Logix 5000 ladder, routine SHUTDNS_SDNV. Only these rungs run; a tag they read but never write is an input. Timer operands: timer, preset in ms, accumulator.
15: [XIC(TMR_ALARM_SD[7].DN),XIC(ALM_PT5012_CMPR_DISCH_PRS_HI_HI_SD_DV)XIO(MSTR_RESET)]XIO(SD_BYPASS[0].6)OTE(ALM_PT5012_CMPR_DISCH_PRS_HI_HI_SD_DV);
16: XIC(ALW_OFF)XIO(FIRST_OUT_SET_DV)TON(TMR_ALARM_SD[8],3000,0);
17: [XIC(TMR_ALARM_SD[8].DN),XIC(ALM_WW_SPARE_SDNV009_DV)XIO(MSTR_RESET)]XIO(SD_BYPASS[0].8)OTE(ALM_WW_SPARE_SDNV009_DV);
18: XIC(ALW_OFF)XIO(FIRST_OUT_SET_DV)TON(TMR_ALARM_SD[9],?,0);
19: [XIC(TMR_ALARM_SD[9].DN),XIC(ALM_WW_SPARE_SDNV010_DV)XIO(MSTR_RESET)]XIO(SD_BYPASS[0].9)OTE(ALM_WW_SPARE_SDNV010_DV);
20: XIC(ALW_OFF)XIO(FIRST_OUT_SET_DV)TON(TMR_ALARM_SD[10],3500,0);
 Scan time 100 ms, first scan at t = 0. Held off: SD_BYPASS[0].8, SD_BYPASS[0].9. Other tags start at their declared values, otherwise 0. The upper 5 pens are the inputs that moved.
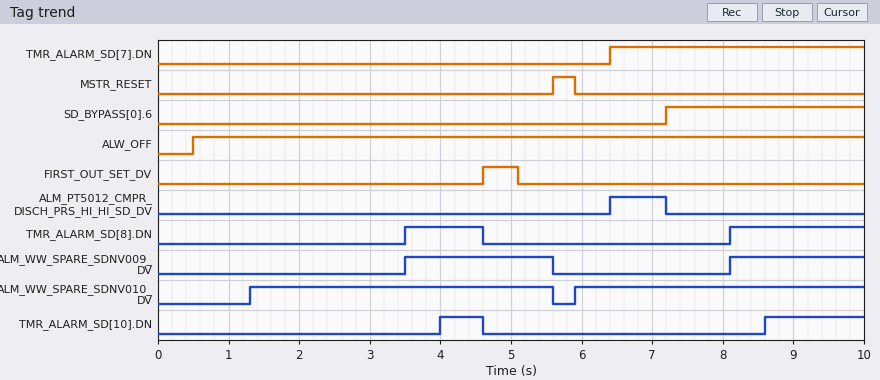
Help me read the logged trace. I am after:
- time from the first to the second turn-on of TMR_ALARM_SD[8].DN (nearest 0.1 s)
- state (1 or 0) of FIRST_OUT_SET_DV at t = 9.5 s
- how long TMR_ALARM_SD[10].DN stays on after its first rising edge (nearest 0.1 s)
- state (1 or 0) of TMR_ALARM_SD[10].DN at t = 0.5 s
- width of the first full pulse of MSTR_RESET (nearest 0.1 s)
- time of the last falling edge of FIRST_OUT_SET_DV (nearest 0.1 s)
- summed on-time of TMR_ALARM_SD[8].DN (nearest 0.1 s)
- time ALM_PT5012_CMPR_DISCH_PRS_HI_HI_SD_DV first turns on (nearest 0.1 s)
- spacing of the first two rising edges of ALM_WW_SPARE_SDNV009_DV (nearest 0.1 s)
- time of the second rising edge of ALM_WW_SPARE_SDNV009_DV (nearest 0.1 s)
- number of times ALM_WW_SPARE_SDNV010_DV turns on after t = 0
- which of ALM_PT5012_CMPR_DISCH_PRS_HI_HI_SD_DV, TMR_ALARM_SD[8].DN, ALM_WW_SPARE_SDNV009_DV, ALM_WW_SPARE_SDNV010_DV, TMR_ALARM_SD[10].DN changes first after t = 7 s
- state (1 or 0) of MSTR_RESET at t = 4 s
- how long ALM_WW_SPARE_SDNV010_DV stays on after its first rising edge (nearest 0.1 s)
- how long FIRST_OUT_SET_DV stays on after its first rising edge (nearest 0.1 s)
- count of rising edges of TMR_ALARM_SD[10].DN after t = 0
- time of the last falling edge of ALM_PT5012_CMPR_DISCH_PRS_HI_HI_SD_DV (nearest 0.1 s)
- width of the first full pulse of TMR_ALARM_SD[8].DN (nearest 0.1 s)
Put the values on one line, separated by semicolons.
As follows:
4.6 s; 0; 0.6 s; 0; 0.3 s; 5.1 s; 3.0 s; 6.4 s; 4.6 s; 8.1 s; 2; ALM_PT5012_CMPR_DISCH_PRS_HI_HI_SD_DV; 0; 4.3 s; 0.5 s; 2; 7.2 s; 1.1 s
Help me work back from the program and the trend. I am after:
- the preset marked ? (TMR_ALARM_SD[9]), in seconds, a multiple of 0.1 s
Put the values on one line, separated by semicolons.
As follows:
0.8 s
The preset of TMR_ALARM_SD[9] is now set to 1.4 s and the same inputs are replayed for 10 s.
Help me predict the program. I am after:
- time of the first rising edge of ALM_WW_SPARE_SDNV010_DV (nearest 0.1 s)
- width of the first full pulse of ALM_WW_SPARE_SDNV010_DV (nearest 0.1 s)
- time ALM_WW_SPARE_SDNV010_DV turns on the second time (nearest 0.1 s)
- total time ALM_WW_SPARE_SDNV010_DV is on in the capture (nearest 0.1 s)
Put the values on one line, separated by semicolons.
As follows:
1.9 s; 3.7 s; 6.5 s; 7.2 s
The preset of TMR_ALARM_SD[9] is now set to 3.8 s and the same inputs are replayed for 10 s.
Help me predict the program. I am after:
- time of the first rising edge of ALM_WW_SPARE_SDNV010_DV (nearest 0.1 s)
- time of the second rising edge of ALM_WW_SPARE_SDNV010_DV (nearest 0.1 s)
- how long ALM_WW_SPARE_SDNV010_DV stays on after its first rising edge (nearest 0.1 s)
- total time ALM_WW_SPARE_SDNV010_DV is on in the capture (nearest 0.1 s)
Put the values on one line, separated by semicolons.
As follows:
4.3 s; 8.9 s; 1.3 s; 2.4 s
